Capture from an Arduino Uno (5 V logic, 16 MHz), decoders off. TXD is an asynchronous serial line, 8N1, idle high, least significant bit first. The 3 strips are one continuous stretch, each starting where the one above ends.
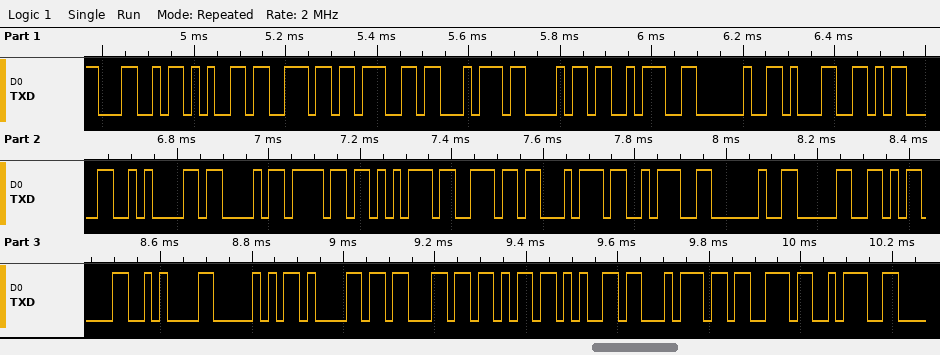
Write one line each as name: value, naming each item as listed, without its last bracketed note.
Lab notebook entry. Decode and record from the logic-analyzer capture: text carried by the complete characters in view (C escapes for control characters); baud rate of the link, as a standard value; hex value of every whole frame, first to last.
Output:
text carried by the complete characters in view: "Length: 1\r\nCount: 0\r\nPackets:"
baud rate of the link, as a standard value: 57600 baud
hex value of every whole frame, first to last: 4C 65 6E 67 74 68 3A 20 31 0D 0A 43 6F 75 6E 74 3A 20 30 0D 0A 50 61 63 6B 65 74 73 3A
